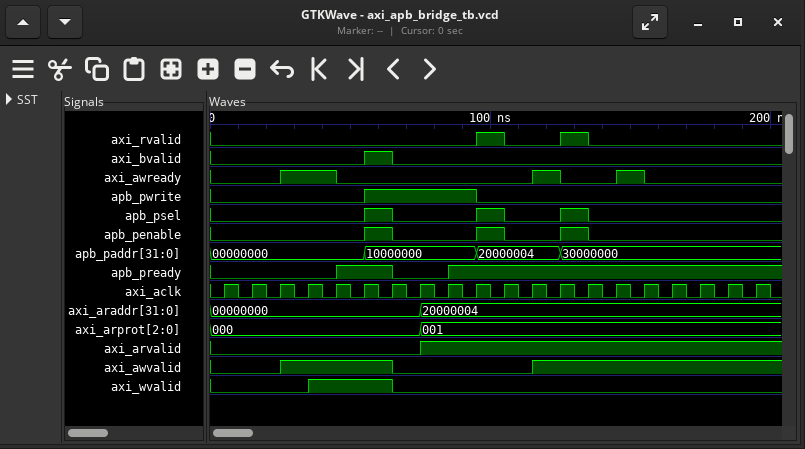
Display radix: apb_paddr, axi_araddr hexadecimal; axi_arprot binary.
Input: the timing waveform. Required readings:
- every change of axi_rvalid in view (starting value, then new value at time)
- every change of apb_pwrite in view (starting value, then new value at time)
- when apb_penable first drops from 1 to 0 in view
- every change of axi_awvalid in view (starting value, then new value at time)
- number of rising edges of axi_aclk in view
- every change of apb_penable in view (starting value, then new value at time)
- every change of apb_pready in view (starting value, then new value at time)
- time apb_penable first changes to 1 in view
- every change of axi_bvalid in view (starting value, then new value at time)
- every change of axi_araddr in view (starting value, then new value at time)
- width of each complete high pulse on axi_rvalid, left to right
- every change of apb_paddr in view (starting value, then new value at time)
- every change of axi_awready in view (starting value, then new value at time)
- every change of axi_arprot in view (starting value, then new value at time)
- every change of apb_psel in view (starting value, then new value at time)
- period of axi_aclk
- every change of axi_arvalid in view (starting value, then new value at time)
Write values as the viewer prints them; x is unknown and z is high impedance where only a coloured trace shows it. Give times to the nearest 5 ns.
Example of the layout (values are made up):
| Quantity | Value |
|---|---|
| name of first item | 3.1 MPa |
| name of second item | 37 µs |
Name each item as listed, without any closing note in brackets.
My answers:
| Quantity | Value |
|---|---|
| every change of axi_rvalid in view | 0, 1 at 95 ns, 0 at 105 ns, 1 at 125 ns, 0 at 135 ns |
| every change of apb_pwrite in view | 0, 1 at 55 ns, 0 at 95 ns |
| when apb_penable first drops from 1 to 0 in view | 65 ns |
| every change of axi_awvalid in view | 0, 1 at 25 ns, 0 at 65 ns, 1 at 115 ns |
| number of rising edges of axi_aclk in view | 20 |
| every change of apb_penable in view | 0, 1 at 55 ns, 0 at 65 ns, 1 at 95 ns, 0 at 105 ns, 1 at 125 ns, 0 at 135 ns |
| every change of apb_pready in view | 0, 1 at 45 ns, 0 at 65 ns, 1 at 85 ns |
| time apb_penable first changes to 1 in view | 55 ns |
| every change of axi_bvalid in view | 0, 1 at 55 ns, 0 at 65 ns |
| every change of axi_araddr in view | 00000000, 20000004 at 75 ns |
| width of each complete high pulse on axi_rvalid, left to right | 10 ns, 10 ns |
| every change of apb_paddr in view | 00000000, 10000000 at 55 ns, 20000004 at 95 ns, 30000000 at 125 ns |
| every change of axi_awready in view | 0, 1 at 25 ns, 0 at 45 ns, 1 at 115 ns, 0 at 125 ns, 1 at 145 ns, 0 at 155 ns |
| every change of axi_arprot in view | 000, 001 at 75 ns |
| every change of apb_psel in view | 0, 1 at 55 ns, 0 at 65 ns, 1 at 95 ns, 0 at 105 ns, 1 at 125 ns, 0 at 135 ns |
| period of axi_aclk | 10 ns |
| every change of axi_arvalid in view | 0, 1 at 75 ns |
